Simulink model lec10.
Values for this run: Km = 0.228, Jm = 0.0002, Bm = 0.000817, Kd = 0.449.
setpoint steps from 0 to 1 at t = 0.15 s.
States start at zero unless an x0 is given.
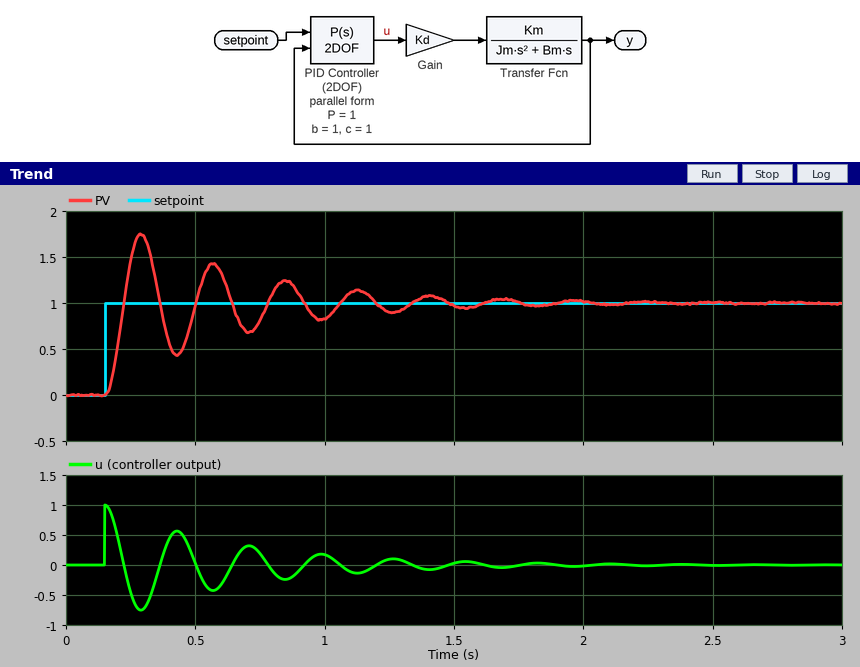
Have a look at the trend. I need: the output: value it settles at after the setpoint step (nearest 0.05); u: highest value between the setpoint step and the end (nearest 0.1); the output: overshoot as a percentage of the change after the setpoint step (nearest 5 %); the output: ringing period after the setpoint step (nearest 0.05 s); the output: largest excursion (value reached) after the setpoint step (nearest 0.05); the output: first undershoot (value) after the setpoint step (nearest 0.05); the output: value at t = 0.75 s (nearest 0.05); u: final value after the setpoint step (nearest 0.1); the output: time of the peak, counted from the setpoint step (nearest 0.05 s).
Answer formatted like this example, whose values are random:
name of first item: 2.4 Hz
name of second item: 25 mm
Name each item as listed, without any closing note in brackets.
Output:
the output: value it settles at after the setpoint step: 1.00
u: highest value between the setpoint step and the end: 1.0
the output: overshoot as a percentage of the change after the setpoint step: 75 %
the output: ringing period after the setpoint step: 0.30 s
the output: largest excursion (value reached) after the setpoint step: 1.75
the output: first undershoot (value) after the setpoint step: 0.45
the output: value at t = 0.75 s: 0.80
u: final value after the setpoint step: 0.0
the output: time of the peak, counted from the setpoint step: 0.15 s
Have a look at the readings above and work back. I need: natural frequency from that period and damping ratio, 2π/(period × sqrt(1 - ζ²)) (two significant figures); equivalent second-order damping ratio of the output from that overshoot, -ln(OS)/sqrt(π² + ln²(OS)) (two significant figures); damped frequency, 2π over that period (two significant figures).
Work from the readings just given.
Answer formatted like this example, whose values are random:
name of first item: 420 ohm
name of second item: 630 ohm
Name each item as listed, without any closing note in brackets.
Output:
natural frequency from that period and damping ratio, 2π/(period × sqrt(1 - ζ²)): 21 rad/s
equivalent second-order damping ratio of the output from that overshoot, -ln(OS)/sqrt(π² + ln²(OS)): 0.091
damped frequency, 2π over that period: 21 rad/s
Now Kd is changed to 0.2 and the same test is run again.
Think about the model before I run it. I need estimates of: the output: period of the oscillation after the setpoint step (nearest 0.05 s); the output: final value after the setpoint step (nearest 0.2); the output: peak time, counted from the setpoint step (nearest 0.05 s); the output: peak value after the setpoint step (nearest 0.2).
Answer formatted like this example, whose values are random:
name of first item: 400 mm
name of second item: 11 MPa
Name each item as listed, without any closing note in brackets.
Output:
the output: period of the oscillation after the setpoint step: 0.40 s
the output: final value after the setpoint step: 1.0
the output: peak time, counted from the setpoint step: 0.20 s
the output: peak value after the setpoint step: 1.6
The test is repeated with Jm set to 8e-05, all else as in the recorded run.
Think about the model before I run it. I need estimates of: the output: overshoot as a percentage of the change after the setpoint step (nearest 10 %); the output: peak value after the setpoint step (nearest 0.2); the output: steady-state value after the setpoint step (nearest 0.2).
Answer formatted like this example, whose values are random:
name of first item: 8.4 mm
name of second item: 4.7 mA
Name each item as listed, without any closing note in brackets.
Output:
the output: overshoot as a percentage of the change after the setpoint step: 60 %
the output: peak value after the setpoint step: 1.6
the output: steady-state value after the setpoint step: 1.0
